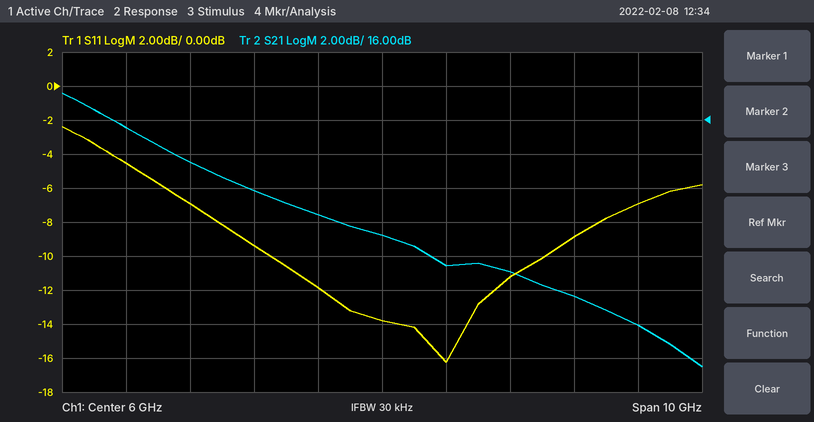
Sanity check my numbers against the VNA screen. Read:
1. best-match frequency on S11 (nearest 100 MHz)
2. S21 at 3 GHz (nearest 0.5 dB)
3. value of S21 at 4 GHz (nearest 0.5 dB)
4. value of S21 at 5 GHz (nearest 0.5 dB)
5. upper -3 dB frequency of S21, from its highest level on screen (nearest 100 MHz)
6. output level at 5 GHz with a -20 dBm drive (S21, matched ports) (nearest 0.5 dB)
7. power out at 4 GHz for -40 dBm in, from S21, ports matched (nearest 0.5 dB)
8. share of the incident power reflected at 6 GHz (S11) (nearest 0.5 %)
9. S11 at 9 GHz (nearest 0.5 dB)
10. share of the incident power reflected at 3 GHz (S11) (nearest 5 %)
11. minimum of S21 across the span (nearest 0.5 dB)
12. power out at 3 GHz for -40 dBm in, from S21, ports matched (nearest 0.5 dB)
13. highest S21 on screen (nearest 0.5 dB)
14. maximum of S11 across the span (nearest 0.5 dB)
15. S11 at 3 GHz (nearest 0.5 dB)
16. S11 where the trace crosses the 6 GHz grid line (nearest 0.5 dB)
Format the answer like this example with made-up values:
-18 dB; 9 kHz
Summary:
7.0 GHz; 13.5 dB; 12.0 dB; 10.5 dB; 2.5 GHz; -9.5 dBm; -28.0 dBm; 4.0 %; -9.0 dB; 20 %; 1.5 dB; -26.5 dBm; 17.5 dB; -2.5 dB; -7.0 dB; -14.0 dB
